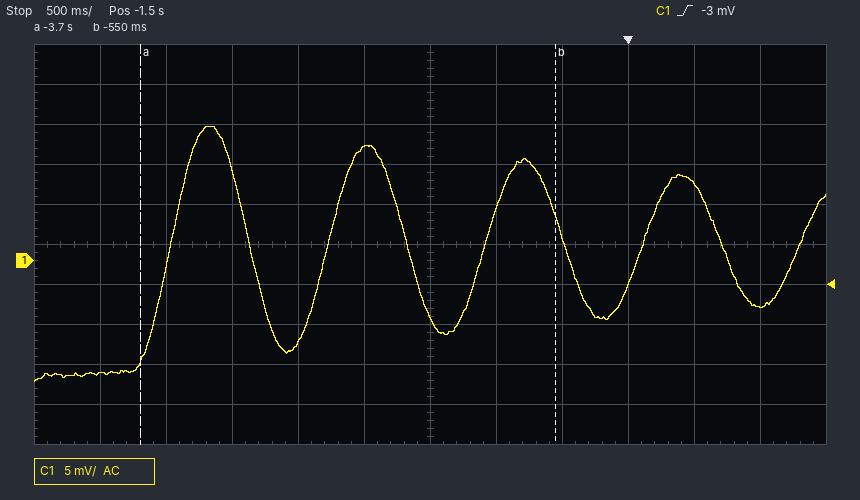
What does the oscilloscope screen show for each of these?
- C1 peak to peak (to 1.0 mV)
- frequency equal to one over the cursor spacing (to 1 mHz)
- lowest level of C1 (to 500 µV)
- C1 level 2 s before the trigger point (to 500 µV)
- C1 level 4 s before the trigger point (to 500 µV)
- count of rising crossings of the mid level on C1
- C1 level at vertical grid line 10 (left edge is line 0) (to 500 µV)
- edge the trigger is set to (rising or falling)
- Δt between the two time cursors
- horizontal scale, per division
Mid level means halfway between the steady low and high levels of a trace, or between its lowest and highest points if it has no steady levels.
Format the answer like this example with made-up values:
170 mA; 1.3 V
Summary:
32.0 mV; 317 mHz; -15.0 mV; 14.0 mV; -14.0 mV; 5; 9.5 mV; rising; 3.15 s; 500 ms
